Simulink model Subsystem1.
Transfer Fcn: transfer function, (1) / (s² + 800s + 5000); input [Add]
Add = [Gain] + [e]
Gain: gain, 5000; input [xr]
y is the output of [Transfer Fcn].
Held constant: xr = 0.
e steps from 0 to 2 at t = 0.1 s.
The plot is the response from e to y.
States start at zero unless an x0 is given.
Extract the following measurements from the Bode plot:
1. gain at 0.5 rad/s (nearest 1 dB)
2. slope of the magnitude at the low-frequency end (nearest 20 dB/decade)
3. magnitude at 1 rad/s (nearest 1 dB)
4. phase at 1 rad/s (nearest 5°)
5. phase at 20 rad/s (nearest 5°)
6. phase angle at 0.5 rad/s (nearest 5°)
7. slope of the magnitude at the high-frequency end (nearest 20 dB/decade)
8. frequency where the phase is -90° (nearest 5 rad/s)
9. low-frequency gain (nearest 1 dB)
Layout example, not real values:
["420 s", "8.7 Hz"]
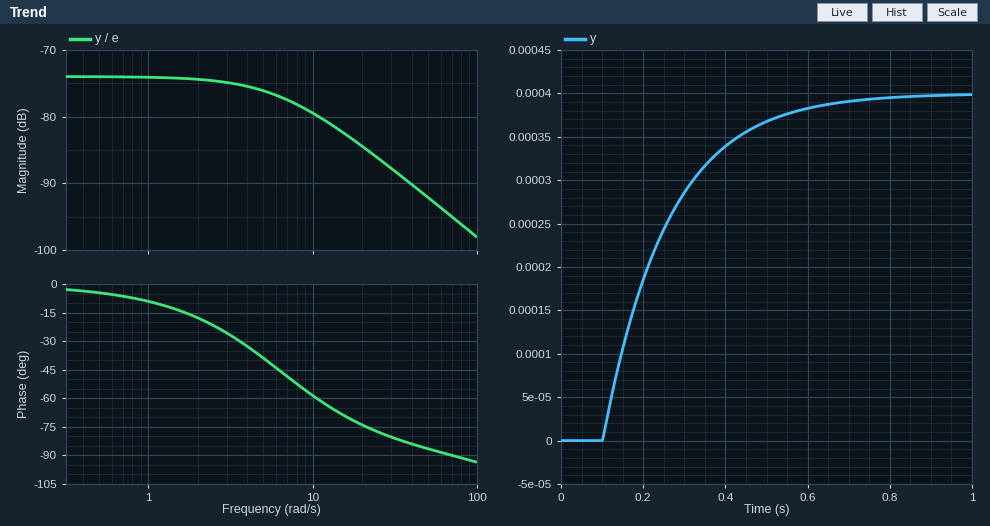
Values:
["-74 dB", "0 dB/decade", "-74 dB", "-10°", "-75°", "-5°", "-20 dB/decade", "70 rad/s", "-74 dB"]
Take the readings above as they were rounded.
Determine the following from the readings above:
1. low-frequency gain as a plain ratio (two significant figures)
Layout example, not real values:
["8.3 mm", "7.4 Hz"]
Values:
["0.00020"]
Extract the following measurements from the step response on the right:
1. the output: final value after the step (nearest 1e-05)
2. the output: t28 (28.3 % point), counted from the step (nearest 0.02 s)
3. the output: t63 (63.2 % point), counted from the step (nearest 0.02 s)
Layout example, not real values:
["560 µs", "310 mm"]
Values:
["0.00040", "0.06 s", "0.16 s"]
